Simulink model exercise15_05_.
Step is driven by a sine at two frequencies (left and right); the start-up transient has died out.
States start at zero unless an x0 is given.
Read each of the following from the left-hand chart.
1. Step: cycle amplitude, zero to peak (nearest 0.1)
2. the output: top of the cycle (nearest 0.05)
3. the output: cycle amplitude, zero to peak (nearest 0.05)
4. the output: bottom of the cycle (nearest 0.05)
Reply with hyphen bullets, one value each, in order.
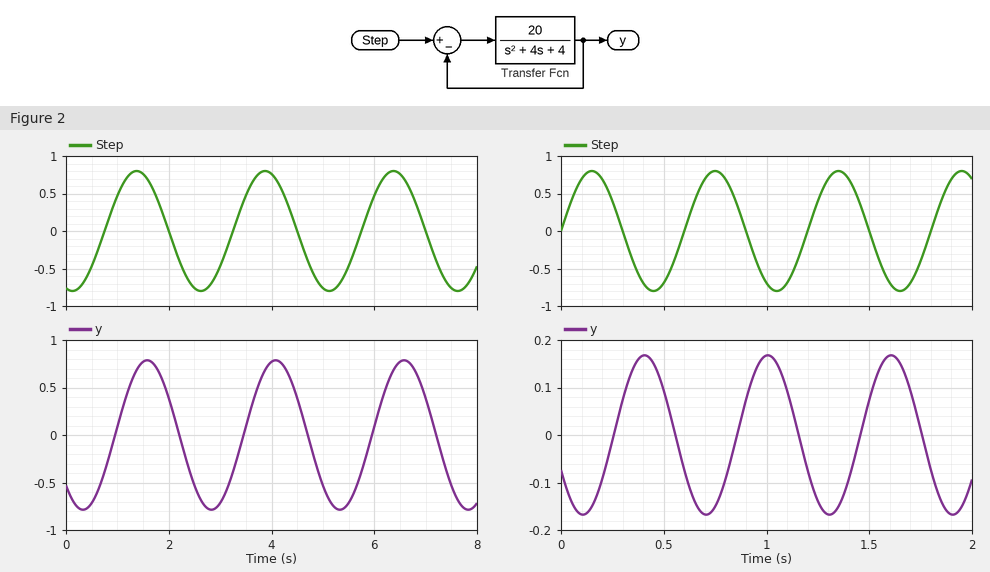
- 0.8
- 0.80
- 0.80
- -0.80
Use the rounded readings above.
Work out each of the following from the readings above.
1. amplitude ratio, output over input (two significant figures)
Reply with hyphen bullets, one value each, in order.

- 1.0
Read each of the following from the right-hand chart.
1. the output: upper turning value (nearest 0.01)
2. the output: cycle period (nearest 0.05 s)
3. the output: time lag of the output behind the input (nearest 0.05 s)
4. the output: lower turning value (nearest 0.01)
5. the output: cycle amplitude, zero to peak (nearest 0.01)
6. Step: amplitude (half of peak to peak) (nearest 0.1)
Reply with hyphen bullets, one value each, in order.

- 0.17
- 0.60 s
- 0.25 s
- -0.17
- 0.17
- 0.8
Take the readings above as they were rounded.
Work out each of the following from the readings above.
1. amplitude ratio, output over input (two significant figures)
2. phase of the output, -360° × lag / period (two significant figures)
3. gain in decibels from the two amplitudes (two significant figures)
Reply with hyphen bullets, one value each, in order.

- 0.21
- -150°
- -13 dB
